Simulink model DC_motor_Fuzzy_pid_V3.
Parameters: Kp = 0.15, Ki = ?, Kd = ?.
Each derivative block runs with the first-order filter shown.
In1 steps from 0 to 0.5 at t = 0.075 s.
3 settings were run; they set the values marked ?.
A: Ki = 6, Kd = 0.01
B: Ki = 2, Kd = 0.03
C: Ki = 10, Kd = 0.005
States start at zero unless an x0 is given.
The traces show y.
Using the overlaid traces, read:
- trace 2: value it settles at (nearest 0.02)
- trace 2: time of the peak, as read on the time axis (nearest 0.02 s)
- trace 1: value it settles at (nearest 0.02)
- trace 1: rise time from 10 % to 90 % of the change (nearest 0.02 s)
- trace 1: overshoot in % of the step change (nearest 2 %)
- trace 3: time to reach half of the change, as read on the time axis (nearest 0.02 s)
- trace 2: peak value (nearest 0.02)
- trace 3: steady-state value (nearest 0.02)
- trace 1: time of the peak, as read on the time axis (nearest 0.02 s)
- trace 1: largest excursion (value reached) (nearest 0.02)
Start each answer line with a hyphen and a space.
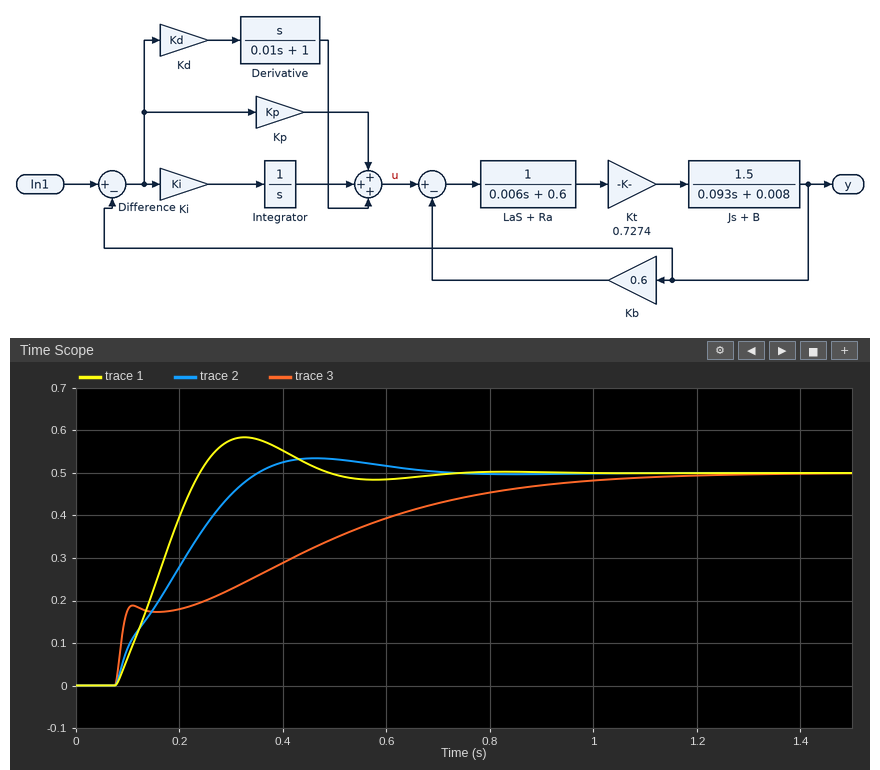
- 0.50
- 0.46 s
- 0.50
- 0.12 s
- 16 %
- 0.34 s
- 0.54
- 0.50
- 0.32 s
- 0.58
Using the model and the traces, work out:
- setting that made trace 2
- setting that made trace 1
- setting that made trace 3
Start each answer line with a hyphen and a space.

- A
- C
- B
